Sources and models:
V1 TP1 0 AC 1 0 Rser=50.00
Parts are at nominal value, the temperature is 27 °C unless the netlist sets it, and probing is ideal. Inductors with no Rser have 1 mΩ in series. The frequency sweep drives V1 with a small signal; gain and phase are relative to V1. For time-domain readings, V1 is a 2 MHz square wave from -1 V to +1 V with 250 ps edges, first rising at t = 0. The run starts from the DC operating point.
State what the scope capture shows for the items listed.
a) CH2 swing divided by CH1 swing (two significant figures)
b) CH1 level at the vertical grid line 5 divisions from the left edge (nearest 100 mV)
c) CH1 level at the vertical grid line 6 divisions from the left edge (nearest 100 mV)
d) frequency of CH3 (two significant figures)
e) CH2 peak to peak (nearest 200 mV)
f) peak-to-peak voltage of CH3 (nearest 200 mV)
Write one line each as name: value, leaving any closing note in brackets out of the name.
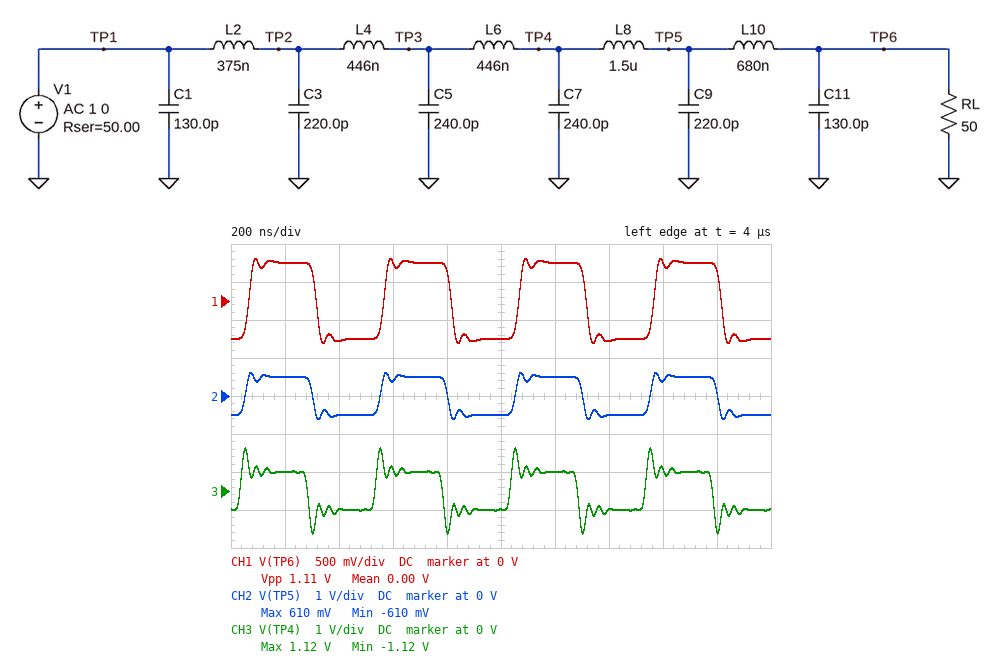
CH2 swing divided by CH1 swing: 1.1
CH1 level at the vertical grid line 5 divisions from the left edge: -500 mV
CH1 level at the vertical grid line 6 divisions from the left edge: 500 mV
frequency of CH3: 2.0 MHz
CH2 peak to peak: 1.2 V
peak-to-peak voltage of CH3: 2.2 V
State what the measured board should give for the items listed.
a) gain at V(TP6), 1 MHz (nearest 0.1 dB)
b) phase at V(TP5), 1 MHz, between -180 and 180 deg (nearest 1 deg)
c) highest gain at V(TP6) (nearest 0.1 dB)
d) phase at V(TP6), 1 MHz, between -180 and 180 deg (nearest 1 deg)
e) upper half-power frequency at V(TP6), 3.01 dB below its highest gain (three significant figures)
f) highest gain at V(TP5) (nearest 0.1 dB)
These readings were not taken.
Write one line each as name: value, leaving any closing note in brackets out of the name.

gain at V(TP6), 1 MHz: -6.0 dB
phase at V(TP5), 1 MHz, between -180 and 180 deg: -18 deg
highest gain at V(TP6): -6.0 dB
phase at V(TP6), 1 MHz, between -180 and 180 deg: -23 deg
upper half-power frequency at V(TP6), 3.01 dB below its highest gain: 16.3 MHz
highest gain at V(TP5): -6.0 dB
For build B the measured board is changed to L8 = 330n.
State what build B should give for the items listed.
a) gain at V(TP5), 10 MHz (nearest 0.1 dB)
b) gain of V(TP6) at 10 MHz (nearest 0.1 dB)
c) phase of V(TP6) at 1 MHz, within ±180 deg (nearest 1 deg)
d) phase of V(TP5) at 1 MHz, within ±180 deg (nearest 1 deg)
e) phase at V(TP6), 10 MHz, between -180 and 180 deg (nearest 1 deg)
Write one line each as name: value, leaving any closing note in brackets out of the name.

gain at V(TP5), 10 MHz: -5.5 dB
gain of V(TP6) at 10 MHz: -6.1 dB
phase of V(TP6) at 1 MHz, within ±180 deg: -19 deg
phase of V(TP5) at 1 MHz, within ±180 deg: -14 deg
phase at V(TP6), 10 MHz, between -180 and 180 deg: 170 deg
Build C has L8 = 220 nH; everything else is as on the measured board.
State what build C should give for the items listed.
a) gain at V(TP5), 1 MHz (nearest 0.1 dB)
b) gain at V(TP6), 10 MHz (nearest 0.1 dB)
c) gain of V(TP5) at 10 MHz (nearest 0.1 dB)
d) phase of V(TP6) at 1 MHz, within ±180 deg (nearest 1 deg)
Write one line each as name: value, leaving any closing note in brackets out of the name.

gain at V(TP5), 1 MHz: -6.0 dB
gain at V(TP6), 10 MHz: -6.1 dB
gain of V(TP5) at 10 MHz: -5.5 dB
phase of V(TP6) at 1 MHz, within ±180 deg: -18 deg
